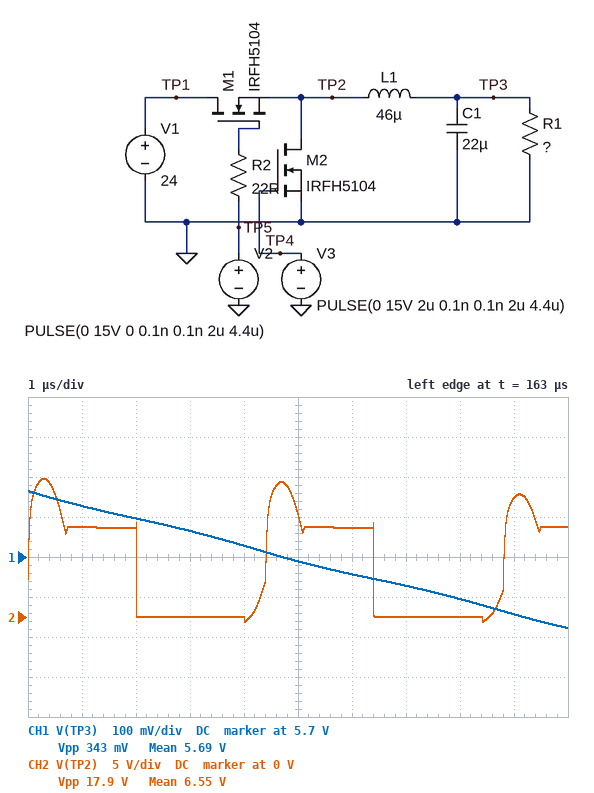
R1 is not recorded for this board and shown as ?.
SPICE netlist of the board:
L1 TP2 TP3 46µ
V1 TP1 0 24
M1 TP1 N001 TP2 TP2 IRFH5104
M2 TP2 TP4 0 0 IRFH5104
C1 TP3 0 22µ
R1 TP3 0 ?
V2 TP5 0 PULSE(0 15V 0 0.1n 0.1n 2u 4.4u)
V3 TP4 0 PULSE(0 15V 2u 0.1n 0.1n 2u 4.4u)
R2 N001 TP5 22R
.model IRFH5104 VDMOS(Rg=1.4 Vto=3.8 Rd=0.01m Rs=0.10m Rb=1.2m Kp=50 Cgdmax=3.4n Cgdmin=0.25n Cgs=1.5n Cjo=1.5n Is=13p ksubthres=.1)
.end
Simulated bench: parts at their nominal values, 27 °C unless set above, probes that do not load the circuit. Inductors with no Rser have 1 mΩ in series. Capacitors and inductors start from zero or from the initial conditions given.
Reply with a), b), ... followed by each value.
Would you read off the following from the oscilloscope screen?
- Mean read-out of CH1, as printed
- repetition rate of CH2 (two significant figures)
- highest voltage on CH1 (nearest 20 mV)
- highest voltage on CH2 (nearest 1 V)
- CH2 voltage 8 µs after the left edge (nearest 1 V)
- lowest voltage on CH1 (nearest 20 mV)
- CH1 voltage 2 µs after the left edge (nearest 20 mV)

a) 5.69 V
b) 230 kHz
c) 5.86 V
d) 17 V
e) 0 V
f) 5.52 V
g) 5.80 V
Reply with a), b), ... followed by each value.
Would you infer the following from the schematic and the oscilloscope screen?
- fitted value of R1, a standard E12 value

a) 6.8 Ω
